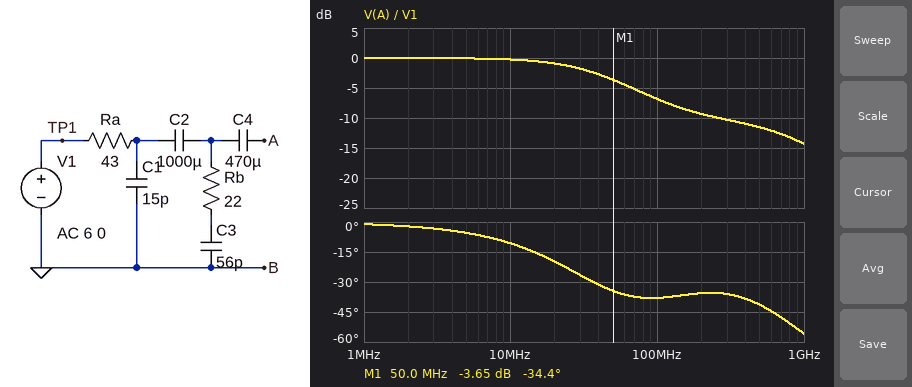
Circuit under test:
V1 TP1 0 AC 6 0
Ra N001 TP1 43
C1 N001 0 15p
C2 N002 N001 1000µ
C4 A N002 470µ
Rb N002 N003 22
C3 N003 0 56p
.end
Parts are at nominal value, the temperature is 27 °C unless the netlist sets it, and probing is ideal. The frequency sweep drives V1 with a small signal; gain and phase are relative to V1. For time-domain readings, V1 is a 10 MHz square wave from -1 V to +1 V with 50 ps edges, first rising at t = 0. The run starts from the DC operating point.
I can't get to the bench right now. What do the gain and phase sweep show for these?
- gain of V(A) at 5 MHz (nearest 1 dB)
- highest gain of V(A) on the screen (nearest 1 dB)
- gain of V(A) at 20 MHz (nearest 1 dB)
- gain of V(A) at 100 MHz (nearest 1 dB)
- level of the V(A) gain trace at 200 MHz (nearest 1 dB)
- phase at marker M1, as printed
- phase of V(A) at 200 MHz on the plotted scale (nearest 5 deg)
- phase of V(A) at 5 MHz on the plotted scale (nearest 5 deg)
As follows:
0 dB
0 dB
-1 dB
-7 dB
-9 dB
-34.4 deg
-35 deg
-5 deg
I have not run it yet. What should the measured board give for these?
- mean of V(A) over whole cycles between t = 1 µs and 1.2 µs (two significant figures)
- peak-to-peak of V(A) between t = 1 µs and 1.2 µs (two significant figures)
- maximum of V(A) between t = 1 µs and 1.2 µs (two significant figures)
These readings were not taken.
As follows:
1.0 V
2.0 V
2.0 V
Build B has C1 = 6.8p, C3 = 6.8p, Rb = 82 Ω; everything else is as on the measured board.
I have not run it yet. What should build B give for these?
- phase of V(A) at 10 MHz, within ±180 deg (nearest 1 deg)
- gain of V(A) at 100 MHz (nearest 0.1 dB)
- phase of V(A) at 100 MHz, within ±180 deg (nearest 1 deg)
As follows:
-2 deg
-0.9 dB
-18 deg
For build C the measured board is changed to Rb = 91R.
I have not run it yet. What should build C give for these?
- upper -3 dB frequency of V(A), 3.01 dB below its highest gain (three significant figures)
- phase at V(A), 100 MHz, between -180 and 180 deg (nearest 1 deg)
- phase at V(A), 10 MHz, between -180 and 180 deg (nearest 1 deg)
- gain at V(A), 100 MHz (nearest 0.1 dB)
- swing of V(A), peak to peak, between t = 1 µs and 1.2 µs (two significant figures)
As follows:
52.8 MHz
-21 deg
-10 deg
-3.7 dB
2.0 V
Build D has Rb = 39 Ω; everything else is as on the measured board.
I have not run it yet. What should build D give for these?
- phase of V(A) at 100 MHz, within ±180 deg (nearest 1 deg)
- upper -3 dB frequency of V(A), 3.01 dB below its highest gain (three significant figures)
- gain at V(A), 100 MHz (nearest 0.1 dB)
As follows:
-28 deg
40.8 MHz
-5.8 dB
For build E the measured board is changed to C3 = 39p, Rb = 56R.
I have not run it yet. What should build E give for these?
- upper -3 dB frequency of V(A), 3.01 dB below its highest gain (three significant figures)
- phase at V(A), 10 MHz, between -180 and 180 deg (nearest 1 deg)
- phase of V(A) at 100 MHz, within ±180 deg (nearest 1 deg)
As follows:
55.6 MHz
-8 deg
-27 deg
